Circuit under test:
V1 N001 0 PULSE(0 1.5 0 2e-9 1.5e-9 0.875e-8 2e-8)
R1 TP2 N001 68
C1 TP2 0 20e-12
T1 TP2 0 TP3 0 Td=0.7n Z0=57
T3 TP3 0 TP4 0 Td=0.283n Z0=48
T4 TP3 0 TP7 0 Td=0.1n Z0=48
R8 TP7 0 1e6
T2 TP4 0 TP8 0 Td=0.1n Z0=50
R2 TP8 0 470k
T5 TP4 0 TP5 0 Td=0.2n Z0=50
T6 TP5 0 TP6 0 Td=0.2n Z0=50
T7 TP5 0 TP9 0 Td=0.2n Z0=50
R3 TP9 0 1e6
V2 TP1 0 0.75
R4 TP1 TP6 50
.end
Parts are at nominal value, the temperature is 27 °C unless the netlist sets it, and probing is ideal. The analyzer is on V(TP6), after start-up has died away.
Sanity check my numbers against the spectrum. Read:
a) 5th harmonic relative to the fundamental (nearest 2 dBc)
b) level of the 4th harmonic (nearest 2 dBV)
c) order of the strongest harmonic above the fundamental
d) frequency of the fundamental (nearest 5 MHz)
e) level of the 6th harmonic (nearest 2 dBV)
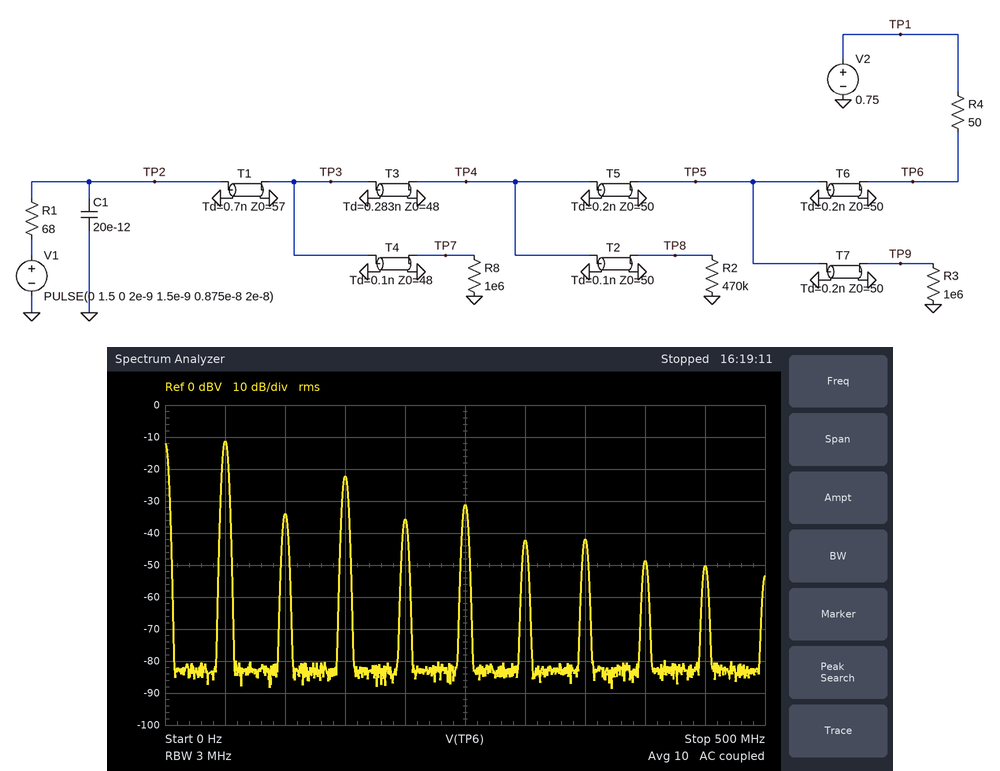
-20 dBc
-36 dBV
3
50 MHz
-42 dBV
